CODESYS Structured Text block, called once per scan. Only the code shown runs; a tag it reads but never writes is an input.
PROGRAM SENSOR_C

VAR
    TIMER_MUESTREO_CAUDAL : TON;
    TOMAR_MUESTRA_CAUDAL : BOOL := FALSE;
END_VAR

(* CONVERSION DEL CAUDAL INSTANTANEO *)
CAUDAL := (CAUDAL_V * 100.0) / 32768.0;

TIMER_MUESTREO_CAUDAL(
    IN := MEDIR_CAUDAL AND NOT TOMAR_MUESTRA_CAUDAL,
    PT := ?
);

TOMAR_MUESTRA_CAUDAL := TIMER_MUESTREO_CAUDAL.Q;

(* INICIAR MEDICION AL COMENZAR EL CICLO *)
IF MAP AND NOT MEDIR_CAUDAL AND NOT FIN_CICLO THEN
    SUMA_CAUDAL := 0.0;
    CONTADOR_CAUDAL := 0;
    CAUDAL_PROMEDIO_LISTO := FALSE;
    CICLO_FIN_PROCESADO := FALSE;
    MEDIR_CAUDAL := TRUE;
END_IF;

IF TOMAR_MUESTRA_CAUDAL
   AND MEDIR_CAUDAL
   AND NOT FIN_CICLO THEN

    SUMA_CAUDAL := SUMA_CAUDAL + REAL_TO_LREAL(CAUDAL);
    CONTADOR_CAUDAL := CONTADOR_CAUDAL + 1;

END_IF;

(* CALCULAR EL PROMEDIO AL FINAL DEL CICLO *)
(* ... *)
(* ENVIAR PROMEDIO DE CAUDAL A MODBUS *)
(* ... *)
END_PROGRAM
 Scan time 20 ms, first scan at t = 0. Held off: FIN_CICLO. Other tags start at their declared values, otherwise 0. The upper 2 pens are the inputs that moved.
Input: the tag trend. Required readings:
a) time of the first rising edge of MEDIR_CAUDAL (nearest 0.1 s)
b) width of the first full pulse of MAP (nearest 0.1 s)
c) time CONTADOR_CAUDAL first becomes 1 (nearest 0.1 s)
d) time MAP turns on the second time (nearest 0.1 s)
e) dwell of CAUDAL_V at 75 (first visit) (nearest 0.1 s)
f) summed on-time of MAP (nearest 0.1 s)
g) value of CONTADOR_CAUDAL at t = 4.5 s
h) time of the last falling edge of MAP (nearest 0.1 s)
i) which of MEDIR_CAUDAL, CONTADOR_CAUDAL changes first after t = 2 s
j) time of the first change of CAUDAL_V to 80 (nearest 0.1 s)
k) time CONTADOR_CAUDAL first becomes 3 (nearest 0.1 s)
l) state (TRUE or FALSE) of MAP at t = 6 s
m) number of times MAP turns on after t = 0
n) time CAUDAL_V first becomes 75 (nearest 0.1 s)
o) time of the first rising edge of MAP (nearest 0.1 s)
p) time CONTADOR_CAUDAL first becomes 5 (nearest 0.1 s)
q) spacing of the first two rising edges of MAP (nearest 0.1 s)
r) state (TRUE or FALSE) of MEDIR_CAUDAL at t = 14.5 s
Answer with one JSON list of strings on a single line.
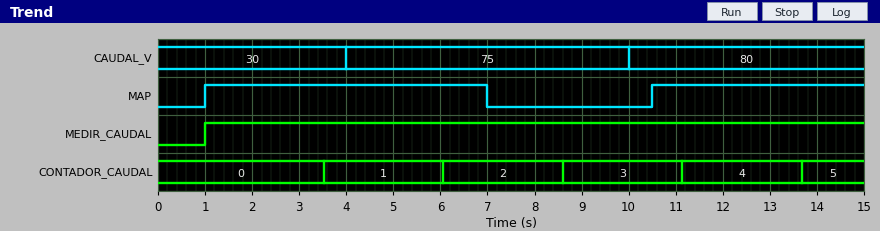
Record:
["1.0 s", "6.0 s", "3.5 s", "10.5 s", "6.0 s", "10.5 s", "1", "7.0 s", "CONTADOR_CAUDAL", "10.0 s", "8.6 s", "TRUE", "2", "4.0 s", "1.0 s", "13.7 s", "9.5 s", "TRUE"]
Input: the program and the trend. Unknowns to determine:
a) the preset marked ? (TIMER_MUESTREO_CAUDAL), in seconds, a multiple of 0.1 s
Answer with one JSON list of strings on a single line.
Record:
["2.5 s"]
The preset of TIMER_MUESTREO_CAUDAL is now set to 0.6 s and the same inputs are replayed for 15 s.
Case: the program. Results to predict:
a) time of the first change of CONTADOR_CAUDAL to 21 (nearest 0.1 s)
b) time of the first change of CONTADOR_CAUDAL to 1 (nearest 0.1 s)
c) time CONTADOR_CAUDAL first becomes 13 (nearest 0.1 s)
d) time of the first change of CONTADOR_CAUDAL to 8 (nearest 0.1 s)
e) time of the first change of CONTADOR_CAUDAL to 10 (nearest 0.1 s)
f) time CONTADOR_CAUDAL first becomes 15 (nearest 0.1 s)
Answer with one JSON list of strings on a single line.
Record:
["14.4 s", "1.6 s", "9.3 s", "6.1 s", "7.4 s", "10.6 s"]
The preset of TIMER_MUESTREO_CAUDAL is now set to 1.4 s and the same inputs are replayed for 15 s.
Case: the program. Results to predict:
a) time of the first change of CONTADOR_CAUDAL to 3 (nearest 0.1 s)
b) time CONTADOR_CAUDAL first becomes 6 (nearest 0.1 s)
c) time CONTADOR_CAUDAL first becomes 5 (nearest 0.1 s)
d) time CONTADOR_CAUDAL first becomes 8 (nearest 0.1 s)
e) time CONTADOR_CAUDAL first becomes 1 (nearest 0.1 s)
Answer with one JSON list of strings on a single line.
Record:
["5.3 s", "9.6 s", "8.2 s", "12.5 s", "2.4 s"]
